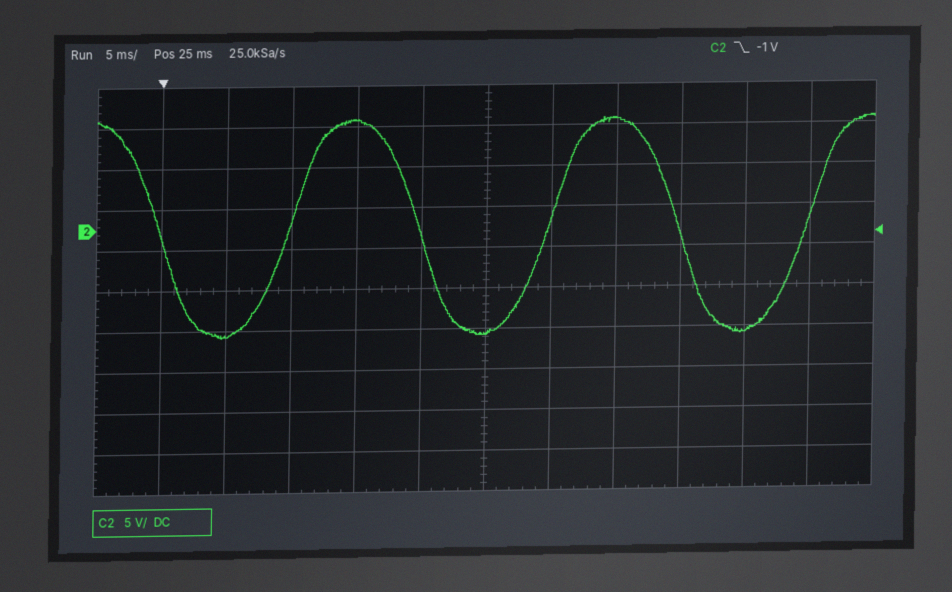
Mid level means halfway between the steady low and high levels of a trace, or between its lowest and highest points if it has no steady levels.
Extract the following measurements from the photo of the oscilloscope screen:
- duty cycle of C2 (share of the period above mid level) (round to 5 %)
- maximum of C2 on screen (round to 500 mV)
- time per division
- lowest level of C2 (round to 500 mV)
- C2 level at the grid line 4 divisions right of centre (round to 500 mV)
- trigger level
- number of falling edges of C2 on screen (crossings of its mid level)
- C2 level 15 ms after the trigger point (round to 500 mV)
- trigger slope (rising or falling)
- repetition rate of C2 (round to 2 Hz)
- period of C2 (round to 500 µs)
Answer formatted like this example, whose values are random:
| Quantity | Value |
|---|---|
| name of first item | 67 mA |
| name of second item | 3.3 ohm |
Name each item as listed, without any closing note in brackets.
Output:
| Quantity | Value |
|---|---|
| duty cycle of C2 (share of the period above mid level) | 50 % |
| maximum of C2 on screen | 13.5 V |
| time per division | 5 ms |
| lowest level of C2 | -13.5 V |
| C2 level at the grid line 4 divisions right of centre | -13.0 V |
| trigger level | -1 V |
| number of falling edges of C2 on screen | 3 |
| C2 level 15 ms after the trigger point | 13.5 V |
| trigger slope | falling |
| repetition rate of C2 | 50 Hz |
| period of C2 | 20.0 ms |
